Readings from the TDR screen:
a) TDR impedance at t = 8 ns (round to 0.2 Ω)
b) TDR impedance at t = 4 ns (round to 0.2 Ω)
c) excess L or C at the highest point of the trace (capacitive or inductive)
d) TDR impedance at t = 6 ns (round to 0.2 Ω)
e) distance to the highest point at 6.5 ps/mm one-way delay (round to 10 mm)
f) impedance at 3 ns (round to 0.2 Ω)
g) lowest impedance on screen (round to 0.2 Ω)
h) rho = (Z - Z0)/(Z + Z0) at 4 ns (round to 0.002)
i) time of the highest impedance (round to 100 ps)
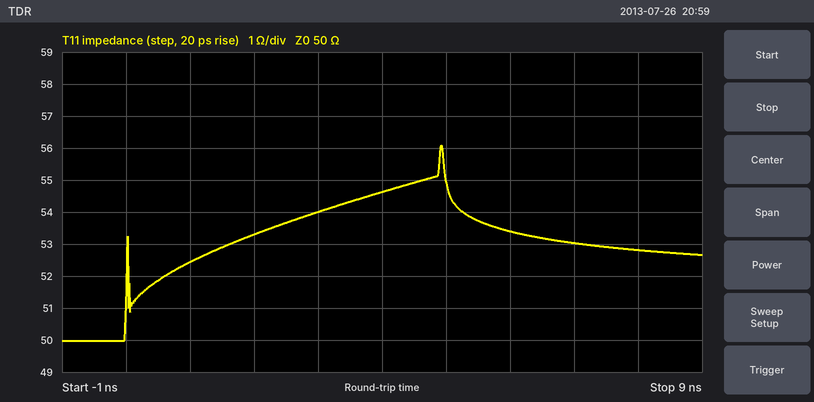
52.8 Ω
54.6 Ω
inductive
53.4 Ω
380 mm
54.0 Ω
50.0 Ω
+0.044
4.9 ns
